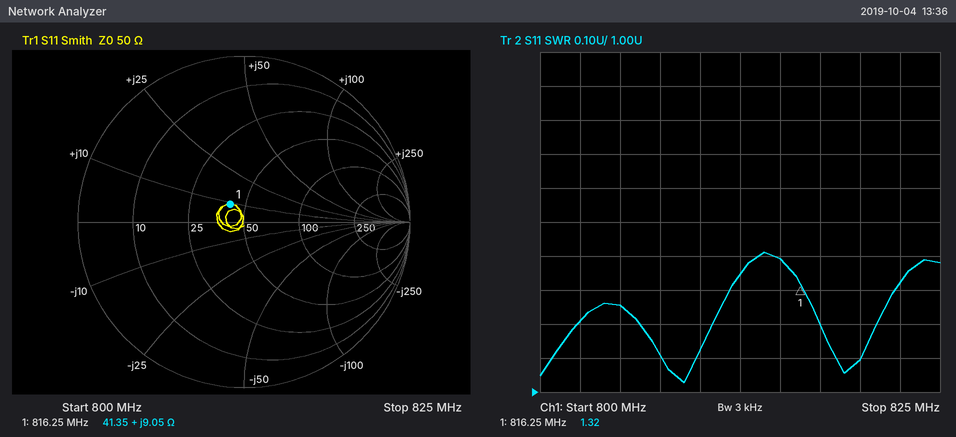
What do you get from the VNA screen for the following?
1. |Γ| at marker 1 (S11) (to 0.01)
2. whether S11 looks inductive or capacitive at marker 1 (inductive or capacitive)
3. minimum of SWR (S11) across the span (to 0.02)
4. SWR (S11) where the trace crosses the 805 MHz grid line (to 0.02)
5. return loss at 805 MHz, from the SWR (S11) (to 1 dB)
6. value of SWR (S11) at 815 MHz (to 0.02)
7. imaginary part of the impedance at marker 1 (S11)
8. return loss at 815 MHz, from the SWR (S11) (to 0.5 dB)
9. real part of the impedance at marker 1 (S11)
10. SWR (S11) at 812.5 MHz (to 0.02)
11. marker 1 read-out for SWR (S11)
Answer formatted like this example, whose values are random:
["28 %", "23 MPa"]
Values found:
["0.14", "inductive", "1.02", "1.26", "19 dB", "1.40", "+9.05 Ω", "15.5 dB", "41.35 Ω", "1.34", "1.32"]
